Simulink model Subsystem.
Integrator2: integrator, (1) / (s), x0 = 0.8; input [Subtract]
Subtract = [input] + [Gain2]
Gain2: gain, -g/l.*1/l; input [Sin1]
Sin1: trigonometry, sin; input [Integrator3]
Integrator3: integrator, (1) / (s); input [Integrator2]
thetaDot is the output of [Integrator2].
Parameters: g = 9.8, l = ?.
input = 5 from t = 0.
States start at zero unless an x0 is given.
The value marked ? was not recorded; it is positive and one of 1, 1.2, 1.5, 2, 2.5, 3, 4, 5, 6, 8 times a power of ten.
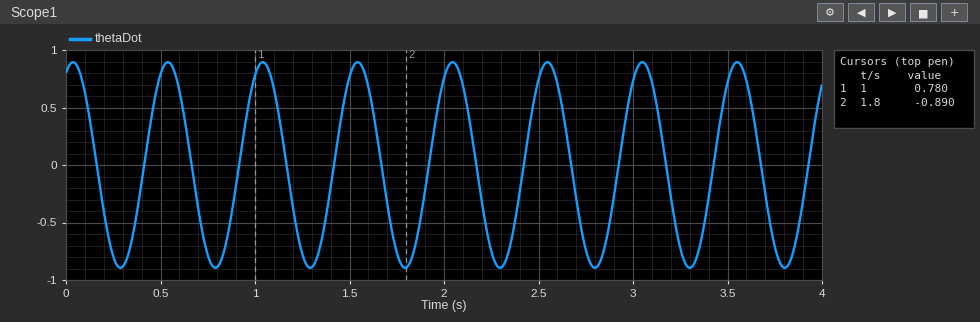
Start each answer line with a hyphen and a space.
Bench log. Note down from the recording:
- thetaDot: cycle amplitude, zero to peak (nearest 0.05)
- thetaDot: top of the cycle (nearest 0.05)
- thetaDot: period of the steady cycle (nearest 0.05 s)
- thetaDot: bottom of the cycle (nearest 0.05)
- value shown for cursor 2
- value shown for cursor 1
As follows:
- 0.90
- 0.90
- 0.50 s
- -0.90
- -0.890
- 0.780
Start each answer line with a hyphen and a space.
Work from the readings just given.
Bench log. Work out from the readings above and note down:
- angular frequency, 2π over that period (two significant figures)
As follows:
- 13 rad/s
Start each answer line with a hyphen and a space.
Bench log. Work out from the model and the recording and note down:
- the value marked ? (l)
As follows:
- 0.25
